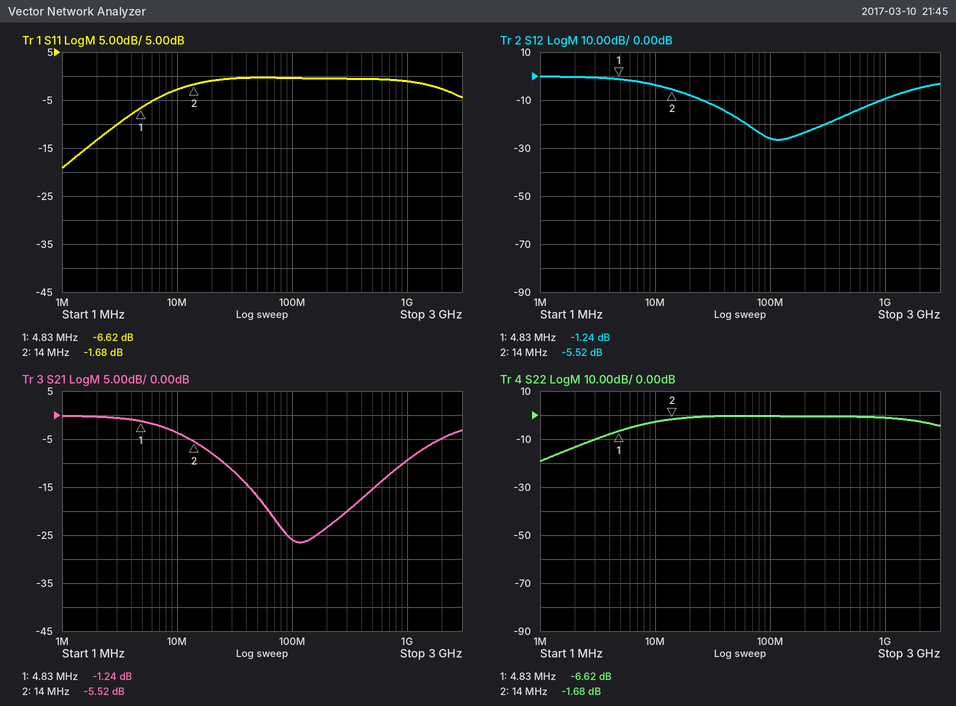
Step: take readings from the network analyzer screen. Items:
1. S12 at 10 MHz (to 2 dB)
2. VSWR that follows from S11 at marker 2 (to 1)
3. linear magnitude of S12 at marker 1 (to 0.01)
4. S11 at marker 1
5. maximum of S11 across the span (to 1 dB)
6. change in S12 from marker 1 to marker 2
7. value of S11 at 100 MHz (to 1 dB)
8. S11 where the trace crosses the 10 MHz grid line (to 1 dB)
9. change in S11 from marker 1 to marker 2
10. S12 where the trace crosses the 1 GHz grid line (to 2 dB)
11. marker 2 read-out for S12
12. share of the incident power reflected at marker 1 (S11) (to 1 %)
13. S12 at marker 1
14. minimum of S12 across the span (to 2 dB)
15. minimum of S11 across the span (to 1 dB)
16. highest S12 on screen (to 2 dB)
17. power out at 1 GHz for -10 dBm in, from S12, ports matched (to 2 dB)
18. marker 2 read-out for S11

-4 dB
10
0.87
-6.62 dB
0 dB
-4.28 dB
0 dB
-3 dB
4.94 dB
-10 dB
-5.52 dB
22 %
-1.24 dB
-26 dB
-19 dB
0 dB
-20 dBm
-1.68 dB
